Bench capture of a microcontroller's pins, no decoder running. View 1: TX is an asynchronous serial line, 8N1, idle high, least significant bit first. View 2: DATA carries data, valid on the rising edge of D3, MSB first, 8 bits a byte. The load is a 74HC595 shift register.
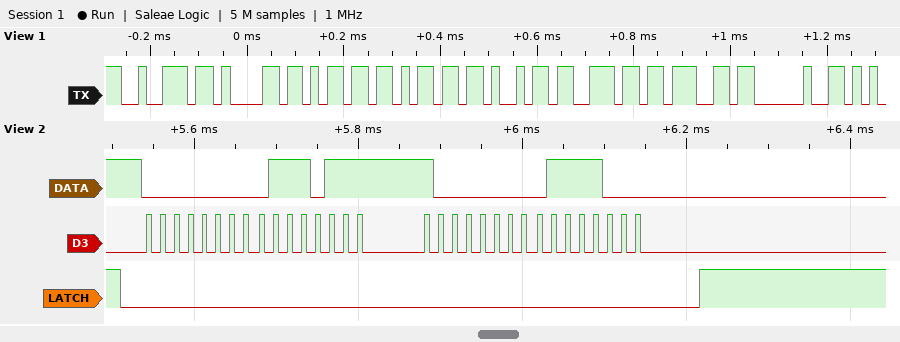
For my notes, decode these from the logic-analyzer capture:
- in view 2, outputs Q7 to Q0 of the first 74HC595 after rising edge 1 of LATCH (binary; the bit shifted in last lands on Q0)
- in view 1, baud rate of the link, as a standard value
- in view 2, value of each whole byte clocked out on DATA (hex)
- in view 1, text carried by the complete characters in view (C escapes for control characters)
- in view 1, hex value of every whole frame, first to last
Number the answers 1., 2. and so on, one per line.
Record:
1. 01111000
2. 57600 baud
3. 00 77 80 78
4. "ramming "
5. 72 61 6D 6D 69 6E 67 20
